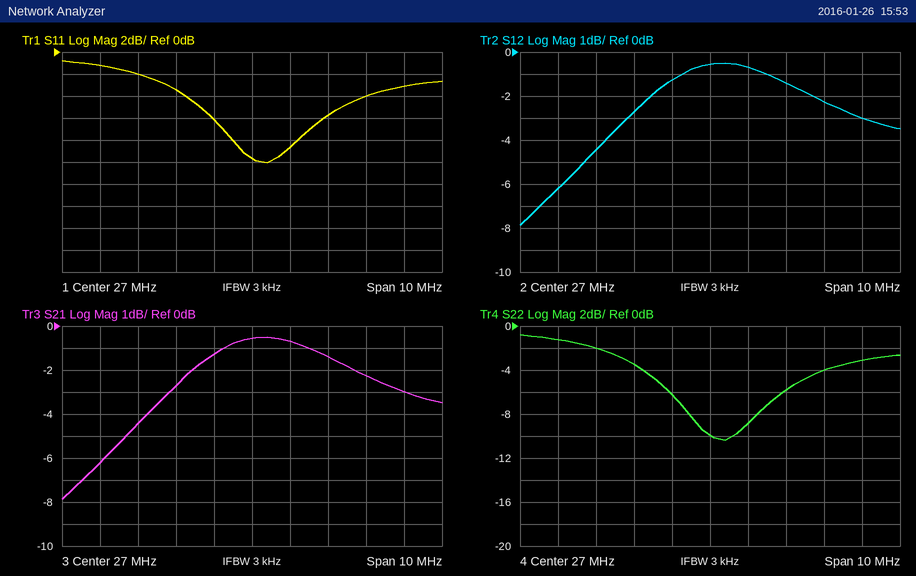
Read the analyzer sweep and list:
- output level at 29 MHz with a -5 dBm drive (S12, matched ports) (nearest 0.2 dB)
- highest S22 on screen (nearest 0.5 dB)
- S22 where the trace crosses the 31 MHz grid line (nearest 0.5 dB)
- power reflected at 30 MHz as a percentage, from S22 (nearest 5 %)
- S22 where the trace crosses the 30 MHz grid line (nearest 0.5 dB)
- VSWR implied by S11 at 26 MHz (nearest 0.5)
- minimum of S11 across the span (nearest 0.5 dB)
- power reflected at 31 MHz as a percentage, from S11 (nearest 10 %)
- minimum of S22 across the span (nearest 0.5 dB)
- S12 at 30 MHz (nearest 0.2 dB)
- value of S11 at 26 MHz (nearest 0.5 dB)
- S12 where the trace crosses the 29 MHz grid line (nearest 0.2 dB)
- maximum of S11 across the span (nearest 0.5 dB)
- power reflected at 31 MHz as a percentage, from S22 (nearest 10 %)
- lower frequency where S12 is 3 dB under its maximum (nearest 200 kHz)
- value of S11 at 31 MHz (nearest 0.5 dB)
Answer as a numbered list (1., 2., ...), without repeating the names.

1. -6.4 dBm
2. -1.0 dB
3. -3.0 dB
4. 40 %
5. -4.0 dB
6. 3.0
7. -10.0 dB
8. 50 %
9. -10.5 dB
10. -2.2 dB
11. -6.0 dB
12. -1.4 dB
13. -1.0 dB
14. 50 %
15. 24.6 MHz
16. -3.0 dB
